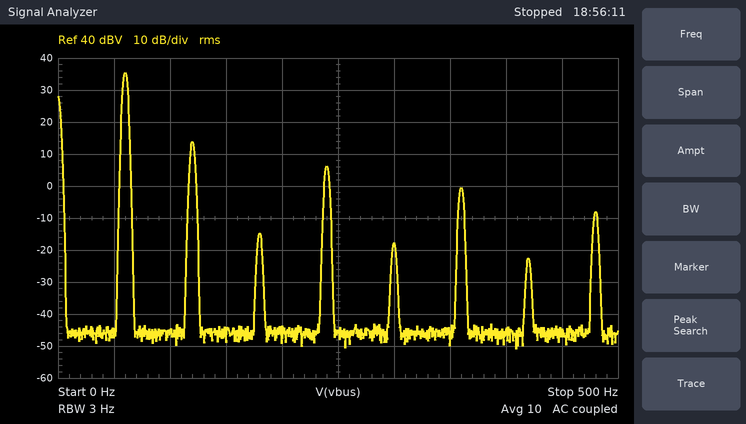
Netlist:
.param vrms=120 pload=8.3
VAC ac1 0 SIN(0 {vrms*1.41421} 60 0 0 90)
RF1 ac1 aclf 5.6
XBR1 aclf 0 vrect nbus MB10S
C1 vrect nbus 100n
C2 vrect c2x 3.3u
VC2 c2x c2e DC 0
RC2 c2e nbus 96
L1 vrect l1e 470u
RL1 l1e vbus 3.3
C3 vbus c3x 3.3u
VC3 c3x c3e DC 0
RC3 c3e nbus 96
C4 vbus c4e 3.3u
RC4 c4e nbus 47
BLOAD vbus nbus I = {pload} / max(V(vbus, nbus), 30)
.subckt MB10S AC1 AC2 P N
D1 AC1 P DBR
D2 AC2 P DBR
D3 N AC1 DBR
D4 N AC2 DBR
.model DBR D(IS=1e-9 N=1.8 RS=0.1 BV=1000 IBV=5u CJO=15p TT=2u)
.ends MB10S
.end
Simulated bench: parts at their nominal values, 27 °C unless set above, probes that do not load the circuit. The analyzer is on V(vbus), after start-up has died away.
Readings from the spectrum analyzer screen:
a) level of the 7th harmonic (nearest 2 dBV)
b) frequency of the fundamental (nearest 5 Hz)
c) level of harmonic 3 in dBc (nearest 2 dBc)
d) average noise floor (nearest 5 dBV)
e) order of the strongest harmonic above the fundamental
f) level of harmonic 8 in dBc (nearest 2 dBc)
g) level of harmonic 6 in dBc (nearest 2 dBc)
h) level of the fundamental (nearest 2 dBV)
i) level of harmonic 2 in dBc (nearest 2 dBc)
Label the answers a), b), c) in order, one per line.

a) -22 dBV
b) 60 Hz
c) -50 dBc
d) -45 dBV
e) 2
f) -44 dBc
g) -36 dBc
h) 36 dBV
i) -22 dBc
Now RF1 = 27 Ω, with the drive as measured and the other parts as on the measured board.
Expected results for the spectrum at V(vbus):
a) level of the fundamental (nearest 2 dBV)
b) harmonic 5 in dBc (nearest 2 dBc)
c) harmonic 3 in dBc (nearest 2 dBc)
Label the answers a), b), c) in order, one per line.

a) 36 dBV
b) -40 dBc
c) -36 dBc
